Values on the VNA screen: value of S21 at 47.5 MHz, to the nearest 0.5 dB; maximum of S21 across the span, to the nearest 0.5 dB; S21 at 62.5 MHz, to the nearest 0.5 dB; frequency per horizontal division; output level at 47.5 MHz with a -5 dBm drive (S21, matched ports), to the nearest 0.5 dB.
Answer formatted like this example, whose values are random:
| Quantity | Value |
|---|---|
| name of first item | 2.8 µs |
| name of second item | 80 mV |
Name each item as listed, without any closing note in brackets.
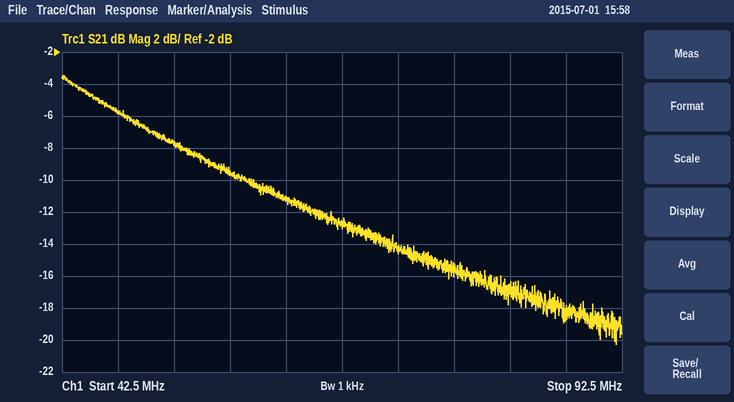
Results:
| Quantity | Value |
|---|---|
| value of S21 at 47.5 MHz, to the nearest 0.5 dB | -6.0 dB |
| maximum of S21 across the span, to the nearest 0.5 dB | -3.5 dB |
| S21 at 62.5 MHz, to the nearest 0.5 dB | -11.0 dB |
| frequency per horizontal division | 5 MHz |
| output level at 47.5 MHz with a -5 dBm drive (S21, matched ports), to the nearest 0.5 dB | -11.0 dBm |
